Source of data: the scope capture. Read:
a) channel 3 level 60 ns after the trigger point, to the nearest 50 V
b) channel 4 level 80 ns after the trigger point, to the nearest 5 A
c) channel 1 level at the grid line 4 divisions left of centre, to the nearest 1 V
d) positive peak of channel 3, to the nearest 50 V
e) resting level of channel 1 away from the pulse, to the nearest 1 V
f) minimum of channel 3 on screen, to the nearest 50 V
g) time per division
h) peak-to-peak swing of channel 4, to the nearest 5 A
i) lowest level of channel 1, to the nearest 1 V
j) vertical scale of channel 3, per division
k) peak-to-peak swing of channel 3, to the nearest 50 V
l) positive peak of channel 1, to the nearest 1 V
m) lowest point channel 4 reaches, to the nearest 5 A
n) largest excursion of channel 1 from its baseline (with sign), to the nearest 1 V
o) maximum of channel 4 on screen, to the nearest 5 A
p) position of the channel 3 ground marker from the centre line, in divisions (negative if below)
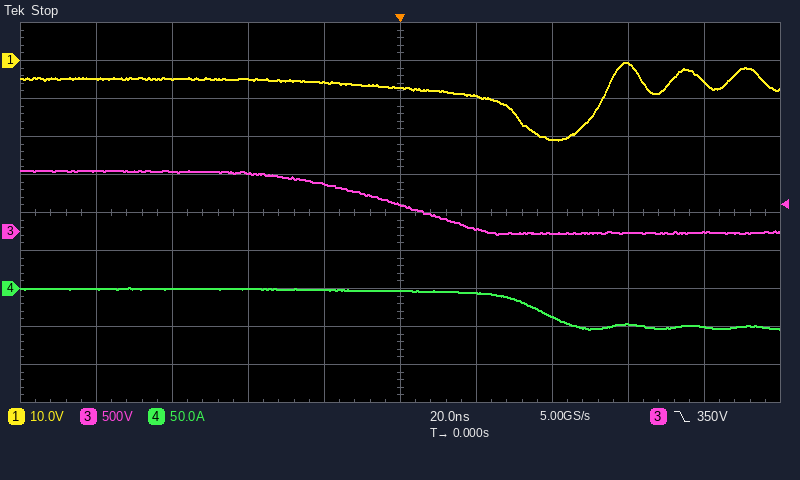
0 V
-50 A
-5 V
800 V
-5 V
-50 V
20 ns
55 A
-21 V
500 V
850 V
-1 V
-55 A
-16 V
0 A
-0.5 div
